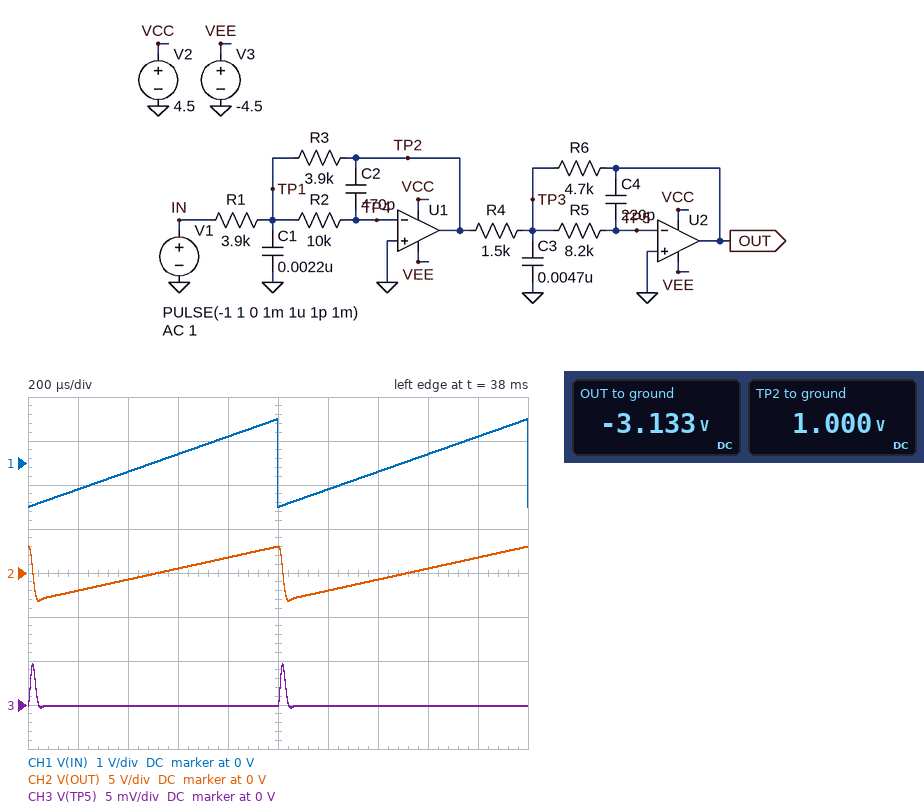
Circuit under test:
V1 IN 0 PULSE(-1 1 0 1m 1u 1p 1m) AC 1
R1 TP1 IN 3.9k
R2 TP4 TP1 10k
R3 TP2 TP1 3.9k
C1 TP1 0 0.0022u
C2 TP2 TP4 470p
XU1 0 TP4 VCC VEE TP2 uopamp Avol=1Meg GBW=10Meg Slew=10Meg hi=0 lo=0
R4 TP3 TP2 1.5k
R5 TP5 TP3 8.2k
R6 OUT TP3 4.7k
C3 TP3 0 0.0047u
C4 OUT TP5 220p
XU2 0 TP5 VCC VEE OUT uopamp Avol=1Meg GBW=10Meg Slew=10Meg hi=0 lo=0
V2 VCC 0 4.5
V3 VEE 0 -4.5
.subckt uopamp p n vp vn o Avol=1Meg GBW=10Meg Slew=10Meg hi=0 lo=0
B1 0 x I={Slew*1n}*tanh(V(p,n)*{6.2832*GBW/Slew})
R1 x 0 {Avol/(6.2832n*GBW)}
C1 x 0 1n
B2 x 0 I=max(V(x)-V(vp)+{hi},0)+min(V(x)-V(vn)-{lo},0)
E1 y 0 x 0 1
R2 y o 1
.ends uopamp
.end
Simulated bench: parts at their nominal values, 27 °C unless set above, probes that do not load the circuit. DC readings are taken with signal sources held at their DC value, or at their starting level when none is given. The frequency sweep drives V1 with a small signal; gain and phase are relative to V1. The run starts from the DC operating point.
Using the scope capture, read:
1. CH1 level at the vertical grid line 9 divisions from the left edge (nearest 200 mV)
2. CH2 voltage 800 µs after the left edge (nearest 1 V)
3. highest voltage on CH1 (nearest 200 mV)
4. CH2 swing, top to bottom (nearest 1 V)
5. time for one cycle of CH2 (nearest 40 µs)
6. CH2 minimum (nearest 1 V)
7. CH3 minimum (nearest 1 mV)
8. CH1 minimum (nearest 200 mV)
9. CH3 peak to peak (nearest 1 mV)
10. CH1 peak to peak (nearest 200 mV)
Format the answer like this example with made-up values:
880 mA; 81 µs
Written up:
600 mV; 2 V; 1.0 V; 6 V; 1.00 ms; -3 V; 0 V; -1.0 V; 5 mV; 2.0 V
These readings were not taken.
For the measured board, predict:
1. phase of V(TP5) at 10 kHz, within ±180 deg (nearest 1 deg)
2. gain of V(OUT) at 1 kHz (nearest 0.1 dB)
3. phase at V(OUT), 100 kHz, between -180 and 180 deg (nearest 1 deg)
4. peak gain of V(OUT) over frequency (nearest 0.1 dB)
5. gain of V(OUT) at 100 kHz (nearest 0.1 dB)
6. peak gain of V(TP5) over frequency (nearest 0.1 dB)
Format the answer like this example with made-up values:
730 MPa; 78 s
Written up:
-163 deg; 9.9 dB; 44 deg; 9.9 dB; -38.4 dB; -48.3 dB
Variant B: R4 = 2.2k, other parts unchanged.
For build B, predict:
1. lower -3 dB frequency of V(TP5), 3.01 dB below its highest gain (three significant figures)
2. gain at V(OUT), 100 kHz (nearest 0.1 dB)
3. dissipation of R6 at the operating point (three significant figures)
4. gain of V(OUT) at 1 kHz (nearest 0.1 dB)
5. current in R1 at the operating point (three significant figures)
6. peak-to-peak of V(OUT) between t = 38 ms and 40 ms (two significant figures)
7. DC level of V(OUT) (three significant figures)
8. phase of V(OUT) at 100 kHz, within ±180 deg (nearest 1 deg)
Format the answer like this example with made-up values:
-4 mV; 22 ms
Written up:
11.0 kHz; -41.6 dB; 971 µW; 6.6 dB; 256 µA; 4.4 V; -2.14 V; 40 deg
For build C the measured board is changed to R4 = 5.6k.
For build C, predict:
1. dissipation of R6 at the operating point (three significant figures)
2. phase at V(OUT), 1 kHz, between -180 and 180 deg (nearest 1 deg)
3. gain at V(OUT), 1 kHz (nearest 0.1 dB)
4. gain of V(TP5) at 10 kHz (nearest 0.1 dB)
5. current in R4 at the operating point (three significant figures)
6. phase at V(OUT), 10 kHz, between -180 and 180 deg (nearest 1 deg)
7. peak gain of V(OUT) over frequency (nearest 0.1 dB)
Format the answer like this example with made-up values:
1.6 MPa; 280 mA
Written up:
150 µW; -6 deg; -1.5 dB; -61.3 dB; 179 µA; -58 deg; -1.0 dB
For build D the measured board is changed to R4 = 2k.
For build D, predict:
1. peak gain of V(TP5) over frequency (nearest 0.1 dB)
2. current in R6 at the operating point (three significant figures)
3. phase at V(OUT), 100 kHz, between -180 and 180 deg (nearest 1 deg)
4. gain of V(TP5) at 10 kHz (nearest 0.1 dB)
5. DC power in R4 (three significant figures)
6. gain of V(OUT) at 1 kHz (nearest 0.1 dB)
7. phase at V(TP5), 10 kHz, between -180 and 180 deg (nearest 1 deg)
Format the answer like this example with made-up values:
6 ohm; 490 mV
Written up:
-49.5 dB; 500 µA; 41 deg; -53.0 dB; 500 µW; 7.4 dB; -158 deg
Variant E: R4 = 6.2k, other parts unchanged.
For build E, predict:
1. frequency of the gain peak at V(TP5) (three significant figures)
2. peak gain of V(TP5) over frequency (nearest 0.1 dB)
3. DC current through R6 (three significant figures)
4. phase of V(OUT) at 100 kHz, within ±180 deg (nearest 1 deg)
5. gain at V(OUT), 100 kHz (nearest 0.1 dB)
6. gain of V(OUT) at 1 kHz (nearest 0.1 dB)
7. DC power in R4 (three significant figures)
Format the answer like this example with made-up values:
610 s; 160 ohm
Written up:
22.6 kHz; -55.4 dB; 161 µA; 34 deg; -50.4 dB; -2.4 dB; 161 µW
